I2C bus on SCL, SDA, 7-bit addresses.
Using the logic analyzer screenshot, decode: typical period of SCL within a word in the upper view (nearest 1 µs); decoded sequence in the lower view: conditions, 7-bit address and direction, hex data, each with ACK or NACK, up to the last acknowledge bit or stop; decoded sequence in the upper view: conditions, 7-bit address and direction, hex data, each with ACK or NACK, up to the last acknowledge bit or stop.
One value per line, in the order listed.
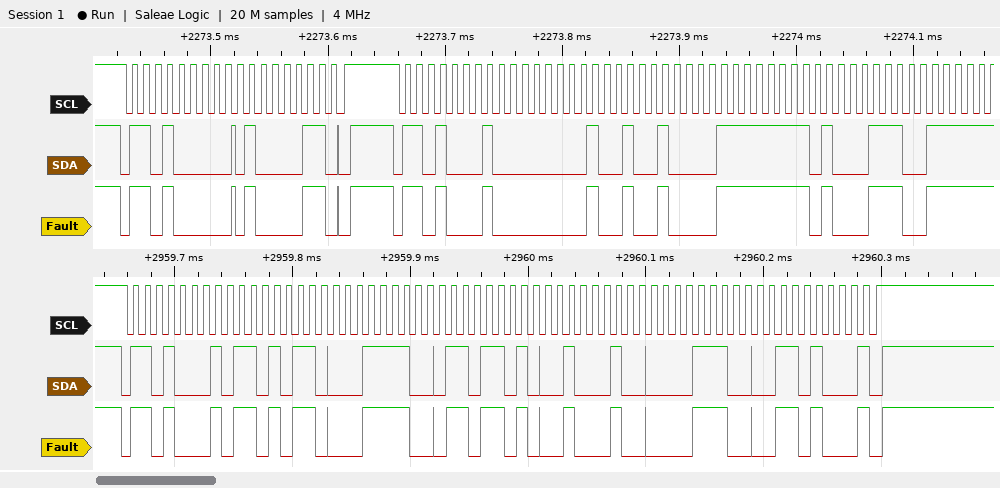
10 µs
start, address 68 read ACK, D6 ACK, 3C ACK, DA ACK, 44 ACK, 1C ACK, 68 NACK, stop
start, address 68 write ACK, 43 ACK, stop, start, address 68 read ACK, 01 ACK, 48 ACK, FF ACK, 8E ACK
